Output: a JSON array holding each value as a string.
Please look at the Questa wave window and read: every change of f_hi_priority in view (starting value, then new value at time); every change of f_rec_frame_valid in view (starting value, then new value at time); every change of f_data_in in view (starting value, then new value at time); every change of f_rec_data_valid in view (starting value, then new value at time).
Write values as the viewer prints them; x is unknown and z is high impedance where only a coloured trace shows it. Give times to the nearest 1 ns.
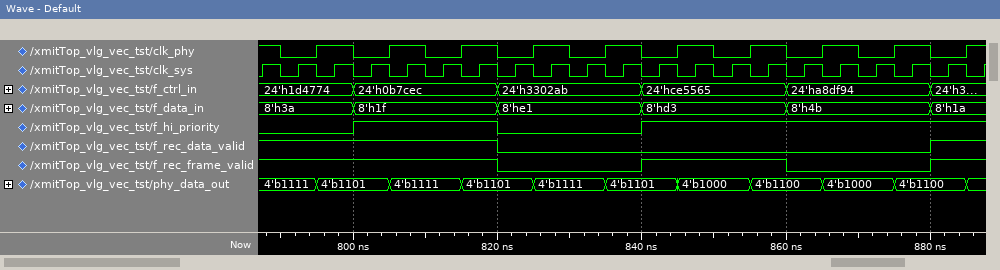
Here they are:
["0, 1 at 800 ns, 0 at 820 ns, 1 at 840 ns", "1, 0 at 820 ns, 1 at 840 ns, 0 at 860 ns, 1 at 880 ns", "8'h3a, 8'h1f at 800 ns, 8'he1 at 820 ns, 8'hd3 at 840 ns, 8'h4b at 860 ns, 8'h1a at 880 ns", "1, 0 at 820 ns, 1 at 880 ns"]
